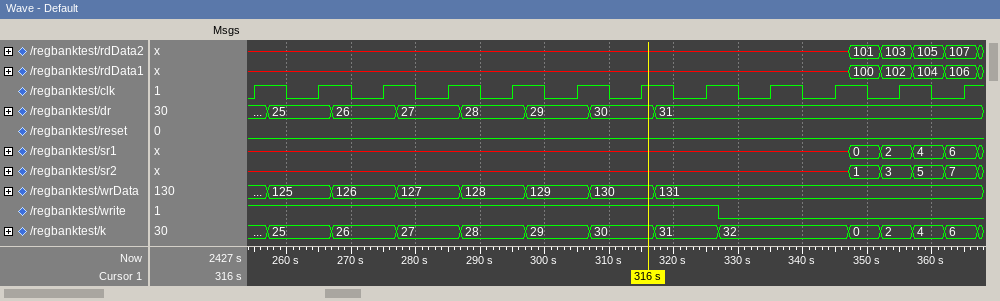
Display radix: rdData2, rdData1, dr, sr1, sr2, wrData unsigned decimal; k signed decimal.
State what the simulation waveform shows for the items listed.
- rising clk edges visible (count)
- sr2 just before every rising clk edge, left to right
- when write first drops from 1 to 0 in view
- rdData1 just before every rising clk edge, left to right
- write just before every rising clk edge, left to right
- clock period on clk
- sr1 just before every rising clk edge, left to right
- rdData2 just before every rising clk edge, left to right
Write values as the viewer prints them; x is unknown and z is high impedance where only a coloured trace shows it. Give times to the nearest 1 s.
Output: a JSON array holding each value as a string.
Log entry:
["12", "x, x, x, x, x, x, x, x, x, x, 3, 7", "327 s", "x, x, x, x, x, x, x, x, x, x, 102, 106", "1 1 1 1 1 1 1 1 0 0 0 0", "10 s", "x, x, x, x, x, x, x, x, x, x, 2, 6", "x, x, x, x, x, x, x, x, x, x, 103, 107"]
